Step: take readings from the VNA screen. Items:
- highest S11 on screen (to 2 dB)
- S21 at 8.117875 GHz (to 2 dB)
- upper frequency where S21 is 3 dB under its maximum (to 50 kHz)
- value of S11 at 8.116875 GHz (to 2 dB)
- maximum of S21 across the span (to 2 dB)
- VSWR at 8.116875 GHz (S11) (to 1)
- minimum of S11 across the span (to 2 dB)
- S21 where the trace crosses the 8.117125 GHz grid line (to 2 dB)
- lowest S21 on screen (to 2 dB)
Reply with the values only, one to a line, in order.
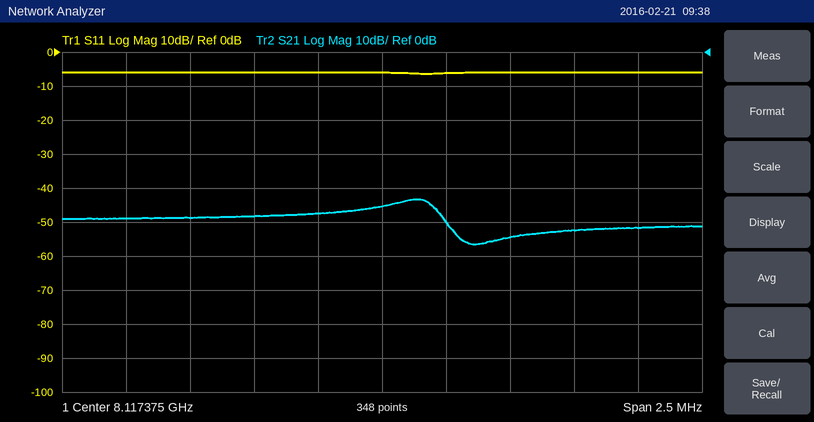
-6 dB
-54 dB
8.11760 GHz
-6 dB
-44 dB
3
-6 dB
-48 dB
-56 dB
